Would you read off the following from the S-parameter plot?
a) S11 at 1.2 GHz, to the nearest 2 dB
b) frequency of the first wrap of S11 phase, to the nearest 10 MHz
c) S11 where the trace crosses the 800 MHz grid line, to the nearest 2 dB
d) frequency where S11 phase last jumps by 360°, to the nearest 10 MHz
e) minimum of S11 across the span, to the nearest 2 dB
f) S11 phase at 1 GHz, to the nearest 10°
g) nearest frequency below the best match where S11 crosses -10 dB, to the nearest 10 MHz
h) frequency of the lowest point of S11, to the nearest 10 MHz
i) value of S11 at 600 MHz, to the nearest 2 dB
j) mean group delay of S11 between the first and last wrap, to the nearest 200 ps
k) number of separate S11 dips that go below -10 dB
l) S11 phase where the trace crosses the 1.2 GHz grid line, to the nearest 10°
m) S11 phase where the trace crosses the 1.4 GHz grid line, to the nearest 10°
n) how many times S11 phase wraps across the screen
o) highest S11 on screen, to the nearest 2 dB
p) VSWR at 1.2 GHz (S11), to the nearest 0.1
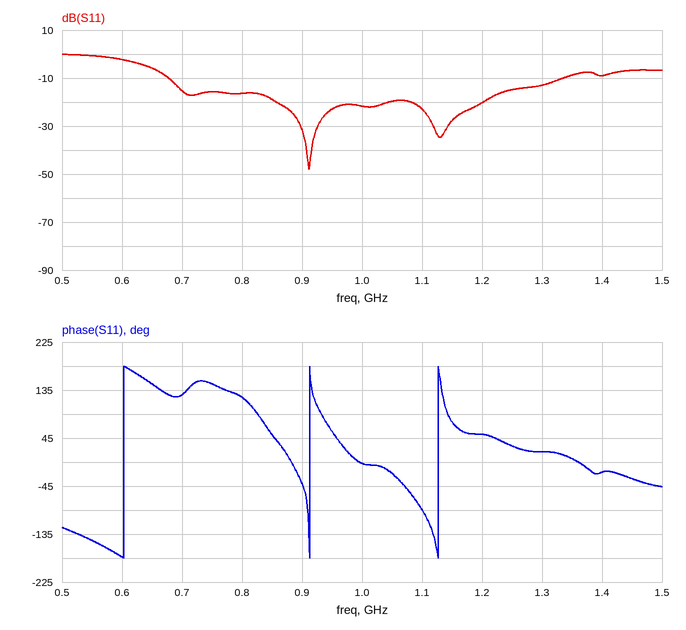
-20 dB
600 MHz
-16 dB
1.13 GHz
-48 dB
0°
680 MHz
910 MHz
-2 dB
3.8 ns
2
50°
-20°
3
0 dB
1.2
